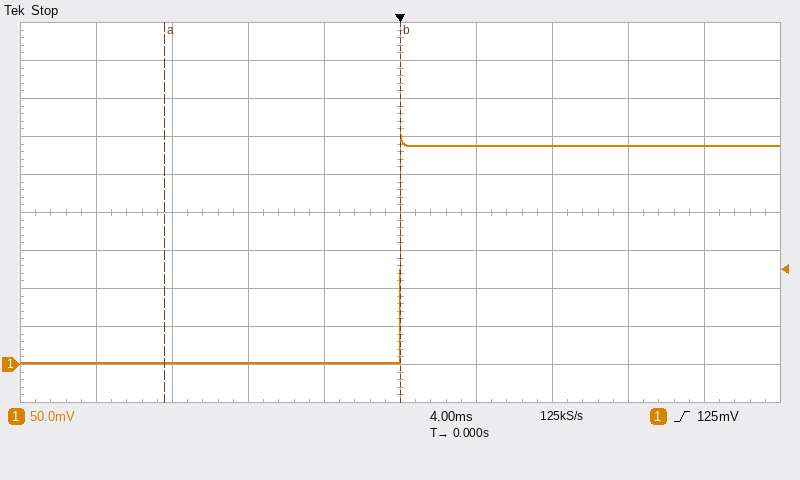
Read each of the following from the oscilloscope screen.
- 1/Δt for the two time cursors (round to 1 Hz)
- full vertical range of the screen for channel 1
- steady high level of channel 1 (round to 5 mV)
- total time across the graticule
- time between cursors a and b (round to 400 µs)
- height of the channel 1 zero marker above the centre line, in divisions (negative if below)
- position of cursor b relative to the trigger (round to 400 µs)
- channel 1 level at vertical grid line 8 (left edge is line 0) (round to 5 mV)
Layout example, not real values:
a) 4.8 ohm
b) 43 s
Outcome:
a) 81 Hz
b) 500 mV
c) 290 mV
d) 40 ms
e) 12.4 ms
f) -4.0 div
g) 0.0 ms
h) 290 mV
